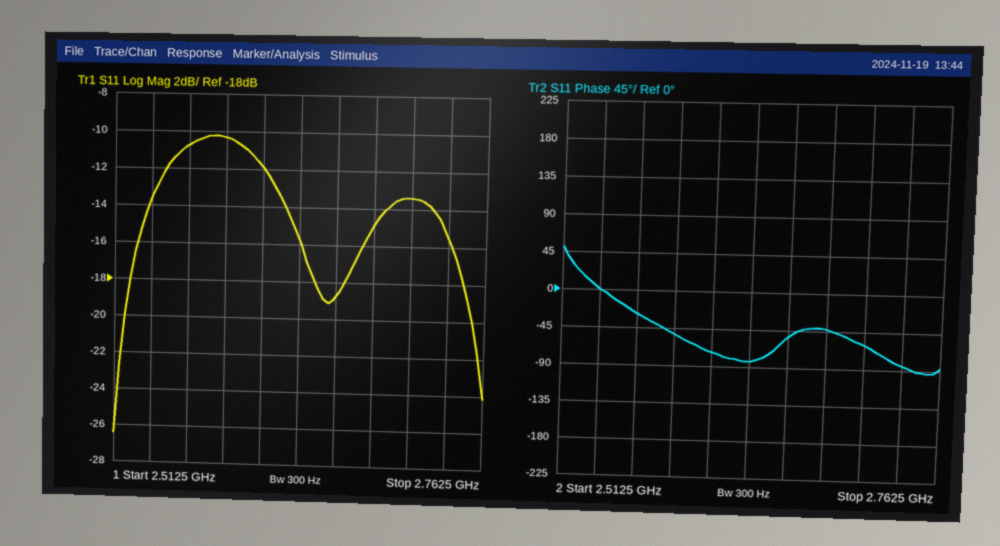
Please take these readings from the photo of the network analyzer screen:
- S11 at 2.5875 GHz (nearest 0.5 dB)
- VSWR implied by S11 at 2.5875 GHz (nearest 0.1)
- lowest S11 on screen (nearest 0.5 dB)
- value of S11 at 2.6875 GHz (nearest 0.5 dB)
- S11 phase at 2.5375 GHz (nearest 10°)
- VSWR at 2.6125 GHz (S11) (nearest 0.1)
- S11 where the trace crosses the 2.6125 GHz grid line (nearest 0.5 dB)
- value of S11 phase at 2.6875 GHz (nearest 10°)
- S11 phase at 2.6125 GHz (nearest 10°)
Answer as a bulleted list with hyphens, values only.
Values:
- -10.5 dB
- 1.9
- -26.5 dB
- -15.0 dB
- 0°
- 1.7
- -12.0 dB
- -40°
- -70°
